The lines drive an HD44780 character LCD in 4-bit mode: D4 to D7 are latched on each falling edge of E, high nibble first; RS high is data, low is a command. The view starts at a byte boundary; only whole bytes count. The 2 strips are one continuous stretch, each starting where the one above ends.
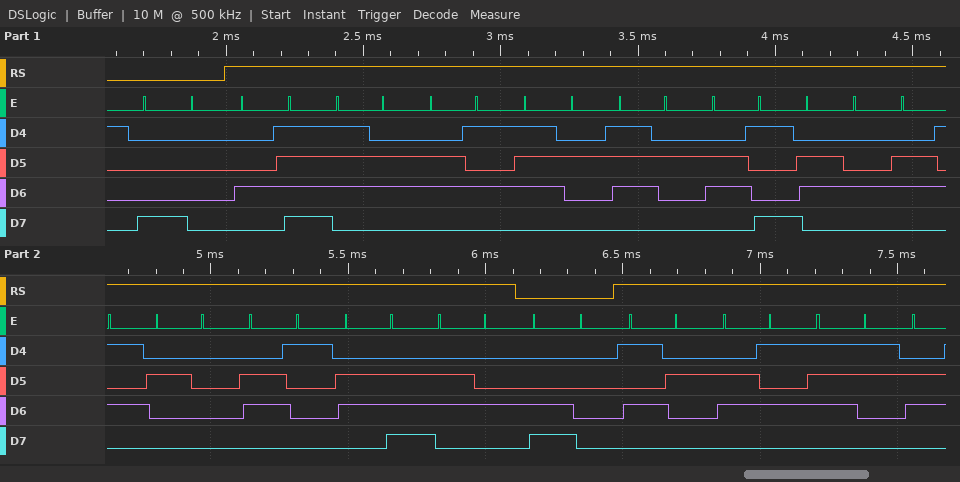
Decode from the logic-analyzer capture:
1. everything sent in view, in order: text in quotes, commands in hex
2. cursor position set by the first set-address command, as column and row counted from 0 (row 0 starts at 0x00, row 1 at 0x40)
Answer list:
0x80 "Override and" 0xC0 "Res"
column 0, row 0
